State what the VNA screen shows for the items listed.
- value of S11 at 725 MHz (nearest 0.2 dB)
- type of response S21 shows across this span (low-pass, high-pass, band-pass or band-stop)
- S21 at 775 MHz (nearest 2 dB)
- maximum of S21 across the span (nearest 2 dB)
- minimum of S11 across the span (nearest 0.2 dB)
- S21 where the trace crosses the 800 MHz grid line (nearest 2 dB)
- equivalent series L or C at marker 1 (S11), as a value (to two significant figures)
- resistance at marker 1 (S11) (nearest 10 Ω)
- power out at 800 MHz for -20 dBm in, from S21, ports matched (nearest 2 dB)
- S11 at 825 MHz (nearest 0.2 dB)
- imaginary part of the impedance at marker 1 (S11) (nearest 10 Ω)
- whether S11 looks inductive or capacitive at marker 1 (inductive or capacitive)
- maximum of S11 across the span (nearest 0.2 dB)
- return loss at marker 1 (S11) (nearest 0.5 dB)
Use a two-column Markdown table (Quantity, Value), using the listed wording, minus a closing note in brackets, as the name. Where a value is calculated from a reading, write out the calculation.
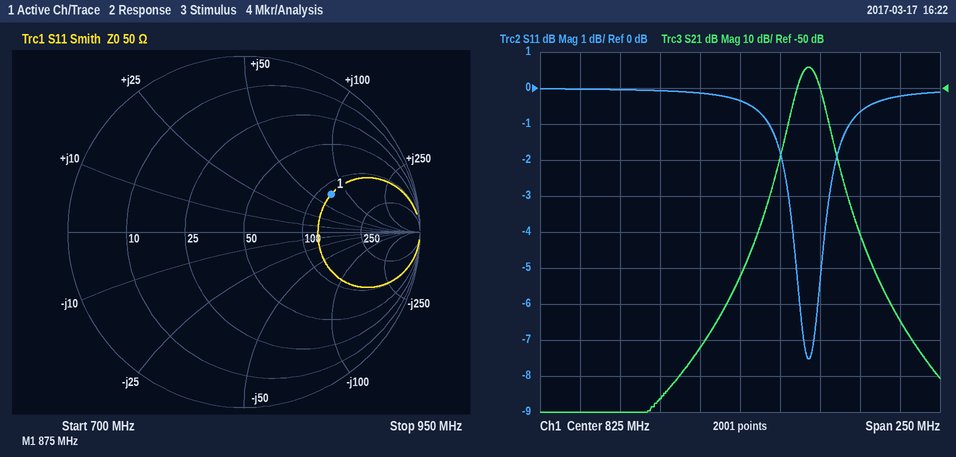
| Quantity | Value |
|---|---|
| value of S11 at 725 MHz | 0.0 dB |
| type of response S21 shows across this span | band-pass |
| S21 at 775 MHz | -136 dB |
| maximum of S21 across the span | -44 dB |
| minimum of S11 across the span | -7.6 dB |
| S21 where the trace crosses the 800 MHz grid line | -122 dB |
| equivalent series L or C at marker 1 (S11), as a value | L = 70 Ω/(2π × 875 MHz) ≈ 13 nH |
| resistance at marker 1 (S11) | 120 Ω |
| power out at 800 MHz for -20 dBm in, from S21, ports matched | -20 dBm + (-122 dB) = -142 dBm |
| S11 at 825 MHz | -0.4 dB |
| imaginary part of the impedance at marker 1 (S11) | +70 Ω |
| whether S11 looks inductive or capacitive at marker 1 | inductive |
| maximum of S11 across the span | 0.0 dB |
| return loss at marker 1 (S11) | 5.5 dB |
